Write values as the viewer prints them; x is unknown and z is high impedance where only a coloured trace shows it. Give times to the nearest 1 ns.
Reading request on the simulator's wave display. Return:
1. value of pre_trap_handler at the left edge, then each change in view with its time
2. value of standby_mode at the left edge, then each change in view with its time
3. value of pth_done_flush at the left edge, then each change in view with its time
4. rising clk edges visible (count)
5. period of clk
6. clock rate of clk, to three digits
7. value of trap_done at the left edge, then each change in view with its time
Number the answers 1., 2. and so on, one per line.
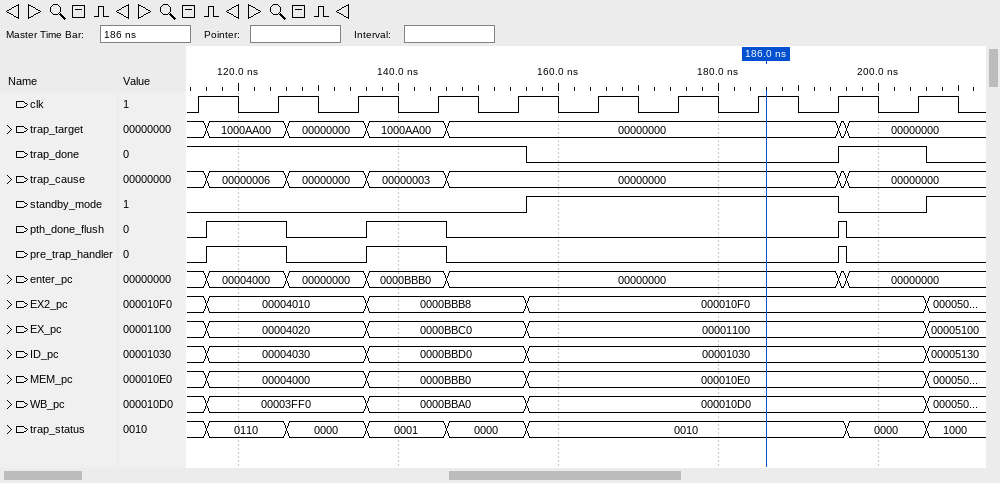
1. 0, 1 at 116 ns, 0 at 126 ns, 1 at 136 ns, 0 at 146 ns, 1 at 195 ns, 0 at 196 ns
2. 0, 1 at 156 ns, 0 at 195 ns, 1 at 206 ns
3. 0, 1 at 116 ns, 0 at 126 ns, 1 at 136 ns, 0 at 146 ns, 1 at 195 ns, 0 at 196 ns
4. 10
5. 10 ns
6. 100 MHz
7. 1, 0 at 156 ns, 1 at 195 ns, 0 at 206 ns
